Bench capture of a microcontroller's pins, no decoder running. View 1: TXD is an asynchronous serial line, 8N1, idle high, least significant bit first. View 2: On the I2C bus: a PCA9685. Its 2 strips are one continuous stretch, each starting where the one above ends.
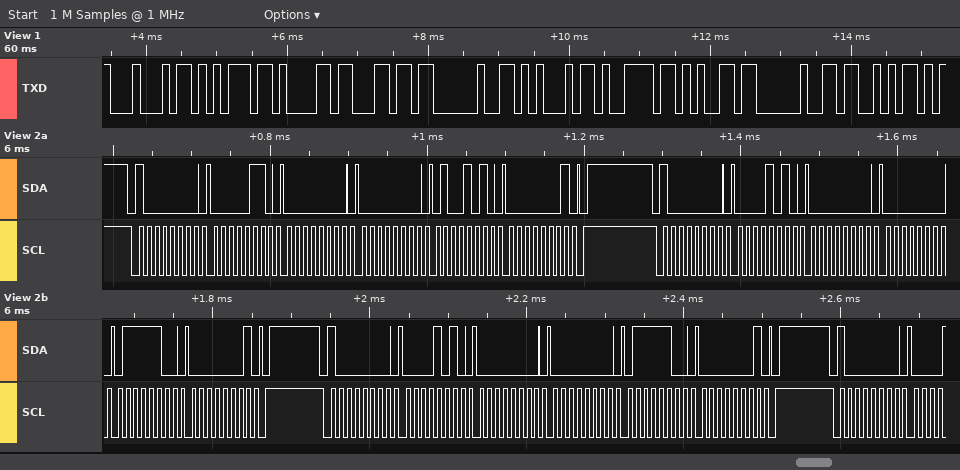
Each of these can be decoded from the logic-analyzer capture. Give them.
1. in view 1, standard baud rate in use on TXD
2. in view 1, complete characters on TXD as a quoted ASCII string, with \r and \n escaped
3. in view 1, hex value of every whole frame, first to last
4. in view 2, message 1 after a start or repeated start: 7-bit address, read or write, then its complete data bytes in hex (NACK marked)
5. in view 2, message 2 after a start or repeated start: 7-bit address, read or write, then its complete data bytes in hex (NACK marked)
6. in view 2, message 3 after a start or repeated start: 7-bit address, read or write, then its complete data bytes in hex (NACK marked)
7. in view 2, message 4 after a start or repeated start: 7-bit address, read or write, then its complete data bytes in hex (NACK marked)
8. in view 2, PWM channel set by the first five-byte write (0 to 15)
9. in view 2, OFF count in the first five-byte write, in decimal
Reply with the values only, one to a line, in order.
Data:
9600 baud
"Dual Eye S"
44 75 61 6C 20 45 79 65 20 53
0x40 write: 06 00 00 4A 01
0x40 write: 0A 00 00 7C 01
0x40 write: 0A 00 00 7C 01
0x40 write
0
330
